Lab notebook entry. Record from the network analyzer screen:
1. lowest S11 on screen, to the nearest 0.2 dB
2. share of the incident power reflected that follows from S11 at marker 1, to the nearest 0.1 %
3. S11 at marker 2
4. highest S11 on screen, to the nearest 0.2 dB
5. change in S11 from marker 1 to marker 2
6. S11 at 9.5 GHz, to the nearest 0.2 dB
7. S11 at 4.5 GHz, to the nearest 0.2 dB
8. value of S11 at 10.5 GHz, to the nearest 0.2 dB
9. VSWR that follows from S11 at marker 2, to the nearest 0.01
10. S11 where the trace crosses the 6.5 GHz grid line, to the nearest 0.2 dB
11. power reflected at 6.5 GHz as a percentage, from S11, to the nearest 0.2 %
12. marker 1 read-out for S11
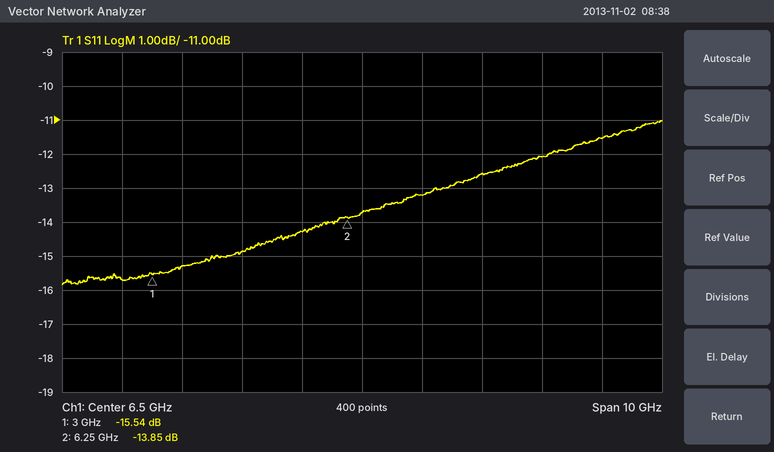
-15.8 dB
2.8 %
-13.85 dB
-11.0 dB
1.69 dB
-12.0 dB
-14.8 dB
-11.6 dB
1.51
-13.8 dB
4.2 %
-15.54 dB
